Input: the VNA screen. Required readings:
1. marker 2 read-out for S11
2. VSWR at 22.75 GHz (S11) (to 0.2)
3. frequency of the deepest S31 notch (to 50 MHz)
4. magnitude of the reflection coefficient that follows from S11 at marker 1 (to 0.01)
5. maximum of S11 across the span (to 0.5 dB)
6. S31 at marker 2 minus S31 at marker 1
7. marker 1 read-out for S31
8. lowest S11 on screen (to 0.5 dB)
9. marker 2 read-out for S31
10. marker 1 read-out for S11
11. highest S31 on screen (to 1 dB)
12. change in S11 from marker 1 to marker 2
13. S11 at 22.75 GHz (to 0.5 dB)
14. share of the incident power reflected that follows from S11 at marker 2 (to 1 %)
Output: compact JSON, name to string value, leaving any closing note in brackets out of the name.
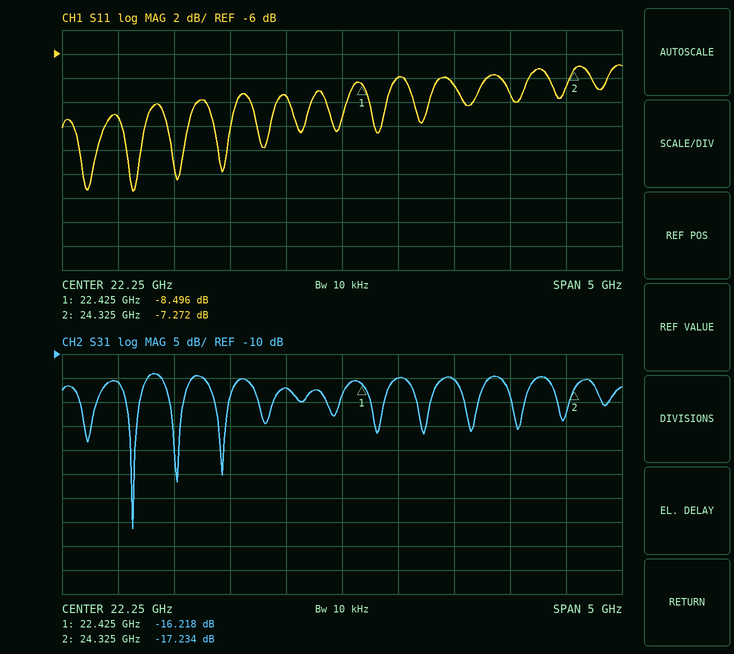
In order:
{"marker 2 read-out for S11": "-7.272 dB", "VSWR at 22.75 GHz (S11)": "2.4", "frequency of the deepest S31 notch": "20.40 GHz", "magnitude of the reflection coefficient that follows from S11 at marker 1": "0.38", "maximum of S11 across the span": "-7.0 dB", "S31 at marker 2 minus S31 at marker 1": "-1.016 dB", "marker 1 read-out for S31": "-16.218 dB", "lowest S11 on screen": "-17.5 dB", "marker 2 read-out for S31": "-17.234 dB", "marker 1 read-out for S11": "-8.496 dB", "highest S31 on screen": "-14 dB", "change in S11 from marker 1 to marker 2": "1.224 dB", "S11 at 22.75 GHz": "-8.0 dB", "share of the incident power reflected that follows from S11 at marker 2": "19 %"}
